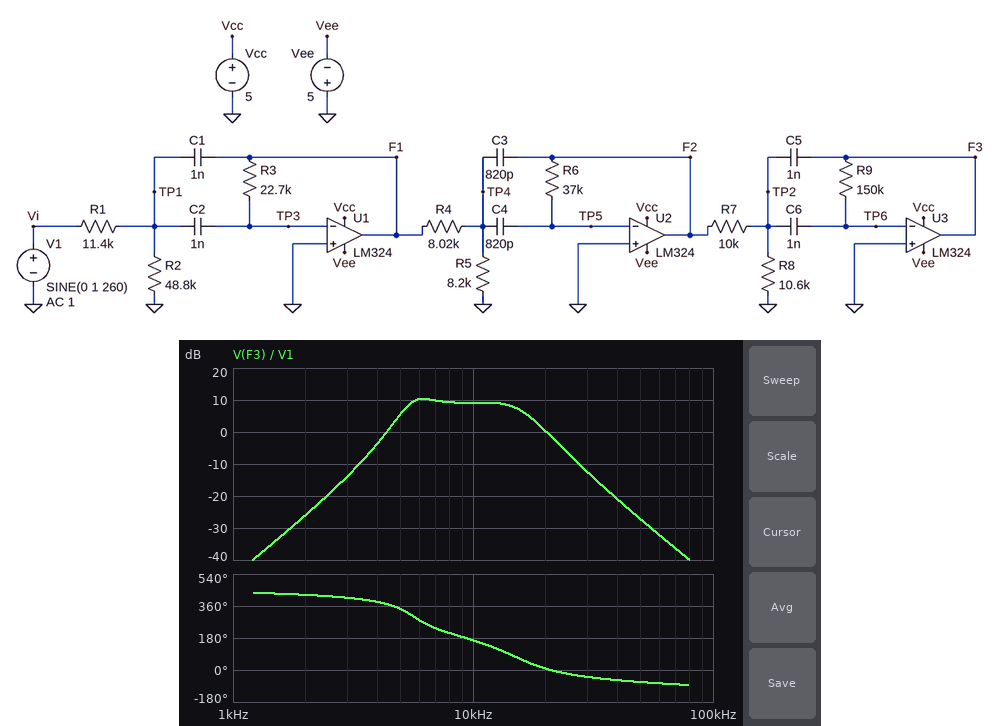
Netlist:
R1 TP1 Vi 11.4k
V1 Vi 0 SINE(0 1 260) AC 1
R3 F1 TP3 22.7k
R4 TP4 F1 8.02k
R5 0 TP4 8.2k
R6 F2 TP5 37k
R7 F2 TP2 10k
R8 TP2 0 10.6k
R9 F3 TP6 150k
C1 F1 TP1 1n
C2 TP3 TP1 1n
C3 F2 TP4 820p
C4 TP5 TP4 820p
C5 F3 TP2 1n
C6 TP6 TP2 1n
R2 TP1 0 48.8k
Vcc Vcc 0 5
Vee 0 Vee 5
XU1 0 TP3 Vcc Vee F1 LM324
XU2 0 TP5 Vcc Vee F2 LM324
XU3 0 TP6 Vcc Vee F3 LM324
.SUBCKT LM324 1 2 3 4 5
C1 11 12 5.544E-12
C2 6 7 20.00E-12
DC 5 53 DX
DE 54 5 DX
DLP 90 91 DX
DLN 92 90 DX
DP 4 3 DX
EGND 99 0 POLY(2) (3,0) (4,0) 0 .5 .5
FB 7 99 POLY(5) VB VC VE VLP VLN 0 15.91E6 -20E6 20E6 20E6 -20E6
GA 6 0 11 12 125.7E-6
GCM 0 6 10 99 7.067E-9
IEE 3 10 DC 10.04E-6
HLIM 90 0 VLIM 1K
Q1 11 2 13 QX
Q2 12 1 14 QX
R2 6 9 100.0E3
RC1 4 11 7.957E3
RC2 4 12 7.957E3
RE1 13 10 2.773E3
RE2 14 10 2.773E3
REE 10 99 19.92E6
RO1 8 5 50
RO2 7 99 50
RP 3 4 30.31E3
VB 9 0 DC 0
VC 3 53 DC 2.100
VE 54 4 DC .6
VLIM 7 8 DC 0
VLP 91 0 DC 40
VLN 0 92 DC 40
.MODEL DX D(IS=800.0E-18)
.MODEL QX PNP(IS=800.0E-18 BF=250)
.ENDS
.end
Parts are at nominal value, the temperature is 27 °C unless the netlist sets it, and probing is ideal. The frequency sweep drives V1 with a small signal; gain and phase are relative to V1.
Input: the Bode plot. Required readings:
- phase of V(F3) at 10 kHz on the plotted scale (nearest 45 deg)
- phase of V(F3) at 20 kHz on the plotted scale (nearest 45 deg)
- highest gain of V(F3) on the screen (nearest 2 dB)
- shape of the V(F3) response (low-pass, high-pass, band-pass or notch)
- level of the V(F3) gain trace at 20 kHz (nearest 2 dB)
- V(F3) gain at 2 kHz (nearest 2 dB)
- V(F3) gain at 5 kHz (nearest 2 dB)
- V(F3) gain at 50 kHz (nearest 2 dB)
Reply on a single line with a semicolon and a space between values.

180 deg; 0 deg; 10 dB; band-pass; 0 dB; -26 dB; 6 dB; -28 dB
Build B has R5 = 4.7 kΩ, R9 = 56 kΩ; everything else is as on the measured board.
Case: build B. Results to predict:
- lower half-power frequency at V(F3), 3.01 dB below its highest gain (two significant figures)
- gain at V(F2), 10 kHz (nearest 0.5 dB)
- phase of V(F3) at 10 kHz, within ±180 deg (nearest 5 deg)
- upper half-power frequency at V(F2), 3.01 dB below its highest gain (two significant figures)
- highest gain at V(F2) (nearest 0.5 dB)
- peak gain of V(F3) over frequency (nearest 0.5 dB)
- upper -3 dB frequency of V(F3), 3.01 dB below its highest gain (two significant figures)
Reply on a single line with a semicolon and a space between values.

8.6 kHz; -0.5 dB; -125 deg; 21 kHz; 5.0 dB; 8.5 dB; 18 kHz
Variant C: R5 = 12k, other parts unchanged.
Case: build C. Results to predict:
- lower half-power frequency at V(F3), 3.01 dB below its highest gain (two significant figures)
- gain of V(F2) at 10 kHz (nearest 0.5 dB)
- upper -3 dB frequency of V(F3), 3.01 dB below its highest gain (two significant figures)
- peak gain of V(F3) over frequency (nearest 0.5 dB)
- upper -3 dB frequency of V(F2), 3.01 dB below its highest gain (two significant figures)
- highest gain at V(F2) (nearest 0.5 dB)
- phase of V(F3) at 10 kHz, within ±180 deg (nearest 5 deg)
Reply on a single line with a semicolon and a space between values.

5.2 kHz; 4.0 dB; 14 kHz; 12.0 dB; 18 kHz; 6.5 dB; 160 deg
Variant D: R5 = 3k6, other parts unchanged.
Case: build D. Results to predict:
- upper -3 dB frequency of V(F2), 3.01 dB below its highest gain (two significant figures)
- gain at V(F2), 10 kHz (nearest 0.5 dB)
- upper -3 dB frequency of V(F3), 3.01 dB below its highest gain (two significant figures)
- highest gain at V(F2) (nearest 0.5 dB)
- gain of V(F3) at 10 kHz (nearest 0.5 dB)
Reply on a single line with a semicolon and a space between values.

23 kHz; -2.5 dB; 20 kHz; 4.5 dB; 4.0 dB
